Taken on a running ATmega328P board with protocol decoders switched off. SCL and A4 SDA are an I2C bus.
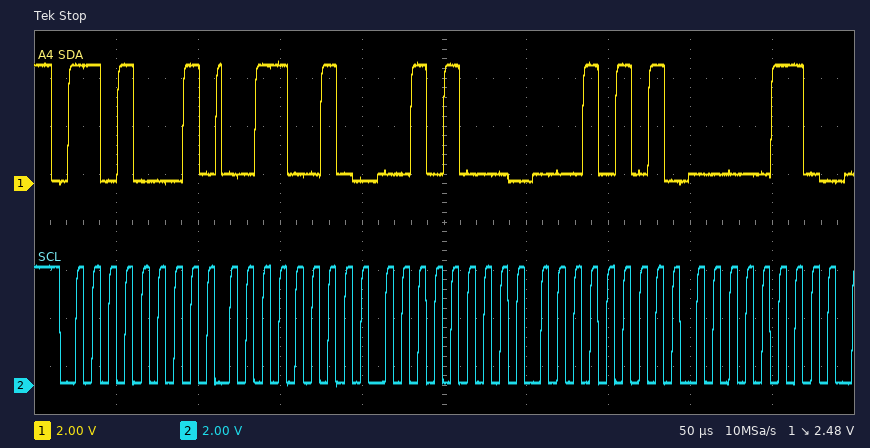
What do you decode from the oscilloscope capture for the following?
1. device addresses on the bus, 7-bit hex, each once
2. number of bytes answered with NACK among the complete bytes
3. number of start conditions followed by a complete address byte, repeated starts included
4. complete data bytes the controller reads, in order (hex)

0x68
0
1
32 28 15 06
